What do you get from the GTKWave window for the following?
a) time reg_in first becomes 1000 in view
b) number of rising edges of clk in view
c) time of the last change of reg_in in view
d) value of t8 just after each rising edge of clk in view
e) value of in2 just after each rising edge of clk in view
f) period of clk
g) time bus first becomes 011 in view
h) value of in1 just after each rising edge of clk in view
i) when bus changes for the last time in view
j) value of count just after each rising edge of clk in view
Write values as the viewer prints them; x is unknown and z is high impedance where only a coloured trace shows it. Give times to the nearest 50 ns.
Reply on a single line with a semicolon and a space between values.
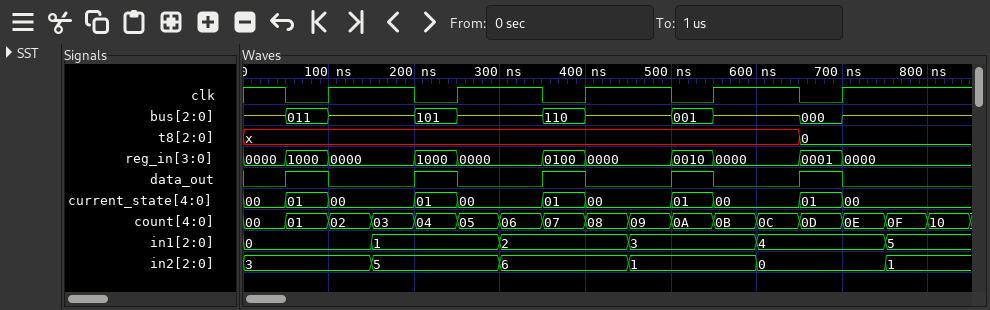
50 ns; 5; 700 ns; x, x, x, x, 0; 3, 5, 6, 1, 0; 150 ns; 50 ns; 0, 1, 2, 3, 4; 700 ns; 02, 05, 08, 0B, 0E
